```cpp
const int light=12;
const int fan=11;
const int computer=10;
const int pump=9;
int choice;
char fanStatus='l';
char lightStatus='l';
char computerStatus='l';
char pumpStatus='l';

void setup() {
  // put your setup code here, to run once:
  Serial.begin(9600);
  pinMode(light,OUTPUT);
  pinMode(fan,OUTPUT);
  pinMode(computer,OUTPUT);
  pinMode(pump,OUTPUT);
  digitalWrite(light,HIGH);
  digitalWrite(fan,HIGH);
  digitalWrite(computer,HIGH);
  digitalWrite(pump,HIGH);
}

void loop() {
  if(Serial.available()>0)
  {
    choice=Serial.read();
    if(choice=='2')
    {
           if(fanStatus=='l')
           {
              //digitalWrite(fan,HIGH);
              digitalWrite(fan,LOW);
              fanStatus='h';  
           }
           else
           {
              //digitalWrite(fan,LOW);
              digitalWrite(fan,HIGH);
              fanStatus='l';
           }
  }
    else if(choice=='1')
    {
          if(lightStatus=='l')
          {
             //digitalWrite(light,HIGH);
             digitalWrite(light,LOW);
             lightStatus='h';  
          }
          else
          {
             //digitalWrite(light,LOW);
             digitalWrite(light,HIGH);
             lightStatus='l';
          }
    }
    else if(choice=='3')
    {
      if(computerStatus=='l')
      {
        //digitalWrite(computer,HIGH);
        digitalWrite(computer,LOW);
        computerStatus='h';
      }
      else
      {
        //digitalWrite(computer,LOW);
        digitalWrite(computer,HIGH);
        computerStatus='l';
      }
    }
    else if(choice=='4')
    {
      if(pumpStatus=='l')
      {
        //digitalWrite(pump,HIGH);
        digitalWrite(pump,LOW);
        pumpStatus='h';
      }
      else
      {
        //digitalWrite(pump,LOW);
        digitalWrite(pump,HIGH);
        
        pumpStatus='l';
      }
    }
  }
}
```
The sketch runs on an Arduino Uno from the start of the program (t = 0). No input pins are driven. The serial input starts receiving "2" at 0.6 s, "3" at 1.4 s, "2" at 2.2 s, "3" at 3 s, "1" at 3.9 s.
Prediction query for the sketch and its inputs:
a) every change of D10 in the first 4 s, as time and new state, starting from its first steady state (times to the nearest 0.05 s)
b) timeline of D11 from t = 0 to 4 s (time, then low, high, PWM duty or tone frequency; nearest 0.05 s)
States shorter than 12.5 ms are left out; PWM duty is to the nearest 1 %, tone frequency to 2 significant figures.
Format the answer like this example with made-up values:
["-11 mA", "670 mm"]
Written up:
["0 s high; 1.4 s low; 3 s high", "0 s high; 0.6 s low; 2.2 s high"]
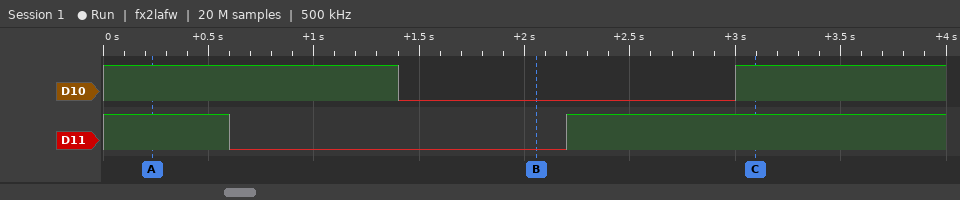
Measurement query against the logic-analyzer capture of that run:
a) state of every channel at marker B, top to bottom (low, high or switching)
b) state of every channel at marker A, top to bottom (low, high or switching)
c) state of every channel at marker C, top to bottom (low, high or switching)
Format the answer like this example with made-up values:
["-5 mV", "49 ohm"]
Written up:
["D10 low, D11 low", "D10 high, D11 high", "D10 high, D11 high"]
